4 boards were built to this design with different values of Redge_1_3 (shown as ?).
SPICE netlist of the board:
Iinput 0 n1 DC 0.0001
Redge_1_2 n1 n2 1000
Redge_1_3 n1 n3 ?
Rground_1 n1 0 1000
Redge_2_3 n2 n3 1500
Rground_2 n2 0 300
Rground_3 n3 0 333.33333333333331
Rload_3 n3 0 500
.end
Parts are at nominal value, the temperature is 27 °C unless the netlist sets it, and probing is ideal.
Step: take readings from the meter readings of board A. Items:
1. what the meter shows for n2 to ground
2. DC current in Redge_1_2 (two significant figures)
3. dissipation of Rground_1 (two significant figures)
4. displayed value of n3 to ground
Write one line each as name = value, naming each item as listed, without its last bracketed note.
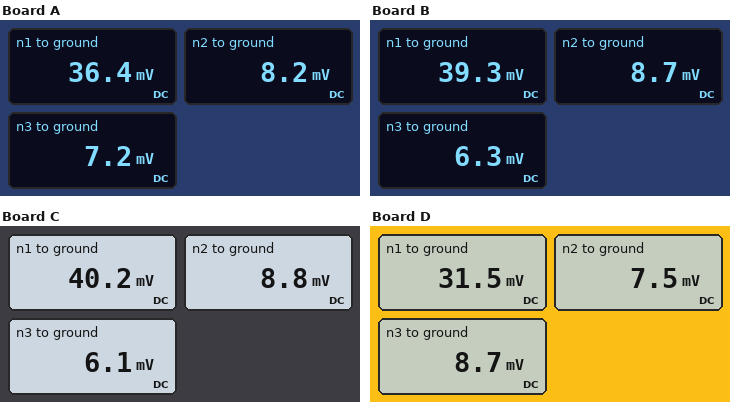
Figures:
what the meter shows for n2 to ground = 8.2 mV
DC current in Redge_1_2 = 28 µA
dissipation of Rground_1 = 1.3 µW
displayed value of n3 to ground = 7.2 mV
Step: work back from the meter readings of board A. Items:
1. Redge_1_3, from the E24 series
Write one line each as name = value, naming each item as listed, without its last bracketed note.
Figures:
Redge_1_3, from the E24 series = 820 Ω
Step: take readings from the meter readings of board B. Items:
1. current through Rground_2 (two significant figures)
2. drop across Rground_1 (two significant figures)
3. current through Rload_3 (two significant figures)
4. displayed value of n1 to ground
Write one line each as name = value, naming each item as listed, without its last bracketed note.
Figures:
current through Rground_2 = 29 µA
drop across Rground_1 = 39 mV
current through Rload_3 = 13 µA
displayed value of n1 to ground = 39.3 mV
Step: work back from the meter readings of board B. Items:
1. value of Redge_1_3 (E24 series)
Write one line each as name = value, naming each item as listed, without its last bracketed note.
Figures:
value of Redge_1_3 = 1.1 kΩ
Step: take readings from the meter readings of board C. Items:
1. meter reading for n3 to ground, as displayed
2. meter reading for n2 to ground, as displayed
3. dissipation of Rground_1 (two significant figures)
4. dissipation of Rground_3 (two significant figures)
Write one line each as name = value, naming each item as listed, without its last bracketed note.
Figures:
meter reading for n3 to ground, as displayed = 6.1 mV
meter reading for n2 to ground, as displayed = 8.8 mV
dissipation of Rground_1 = 1.6 µW
dissipation of Rground_3 = 110 nW
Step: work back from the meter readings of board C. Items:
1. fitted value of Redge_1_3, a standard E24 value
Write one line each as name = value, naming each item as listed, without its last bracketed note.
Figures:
fitted value of Redge_1_3, a standard E24 value = 1.2 kΩ
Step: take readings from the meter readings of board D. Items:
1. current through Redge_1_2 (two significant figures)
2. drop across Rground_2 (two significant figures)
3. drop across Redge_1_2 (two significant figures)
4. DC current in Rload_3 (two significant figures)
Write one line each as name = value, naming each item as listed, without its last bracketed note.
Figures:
current through Redge_1_2 = 24 µA
drop across Rground_2 = 7.5 mV
drop across Redge_1_2 = 24 mV
DC current in Rload_3 = 17 µA
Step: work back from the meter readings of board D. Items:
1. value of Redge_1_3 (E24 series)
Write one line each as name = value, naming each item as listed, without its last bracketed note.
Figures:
value of Redge_1_3 = 510 Ω
